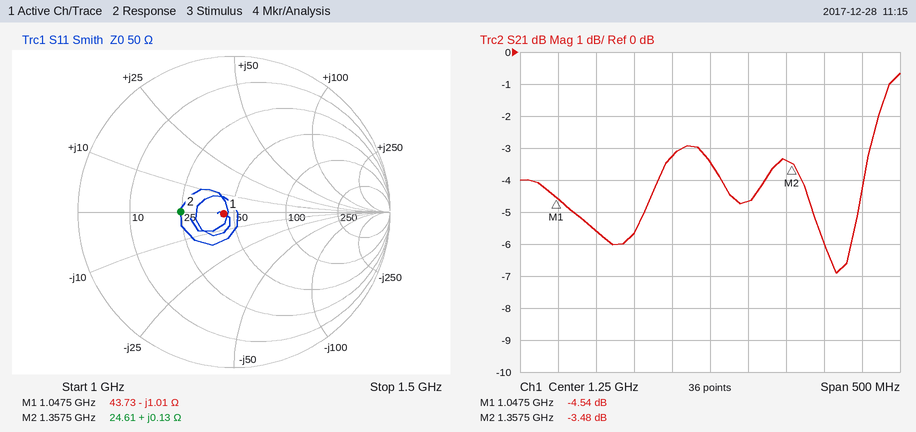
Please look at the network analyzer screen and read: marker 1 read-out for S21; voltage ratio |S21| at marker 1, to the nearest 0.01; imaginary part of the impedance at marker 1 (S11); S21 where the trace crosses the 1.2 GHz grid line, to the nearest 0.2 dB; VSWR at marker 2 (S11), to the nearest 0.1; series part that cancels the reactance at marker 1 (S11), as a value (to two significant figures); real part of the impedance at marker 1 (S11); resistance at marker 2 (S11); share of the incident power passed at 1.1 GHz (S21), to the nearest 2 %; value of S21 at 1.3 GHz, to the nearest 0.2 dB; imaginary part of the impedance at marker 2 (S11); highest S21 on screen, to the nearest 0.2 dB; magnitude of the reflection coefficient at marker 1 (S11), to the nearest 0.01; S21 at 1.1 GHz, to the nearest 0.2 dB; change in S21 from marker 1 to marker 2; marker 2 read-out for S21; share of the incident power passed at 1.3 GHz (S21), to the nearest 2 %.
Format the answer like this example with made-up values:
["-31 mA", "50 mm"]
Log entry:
["-4.54 dB", "0.59", "-1.01 Ω", "-3.2 dB", "2.0", "150 pH", "43.73 Ω", "24.61 Ω", "28 %", "-4.6 dB", "+0.13 Ω", "-0.6 dB", "0.07", "-5.6 dB", "1.06 dB", "-3.48 dB", "34 %"]
